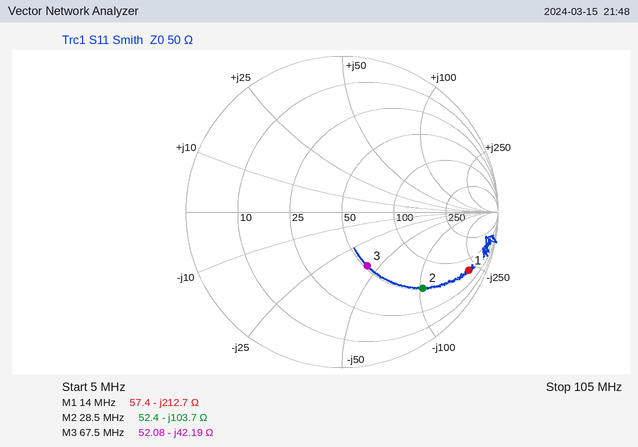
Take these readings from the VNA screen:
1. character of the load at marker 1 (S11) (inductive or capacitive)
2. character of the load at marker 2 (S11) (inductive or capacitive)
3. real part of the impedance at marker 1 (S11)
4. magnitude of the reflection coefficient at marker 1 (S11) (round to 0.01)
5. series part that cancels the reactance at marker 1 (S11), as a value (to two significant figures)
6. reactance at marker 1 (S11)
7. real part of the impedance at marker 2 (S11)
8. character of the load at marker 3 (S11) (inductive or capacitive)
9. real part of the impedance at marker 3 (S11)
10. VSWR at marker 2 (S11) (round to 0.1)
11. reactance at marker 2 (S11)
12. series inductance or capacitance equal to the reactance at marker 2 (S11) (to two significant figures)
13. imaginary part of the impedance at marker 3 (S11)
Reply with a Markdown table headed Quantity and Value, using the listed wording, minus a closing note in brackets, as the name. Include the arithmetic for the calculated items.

| Quantity | Value |
|---|---|
| character of the load at marker 1 (S11) | capacitive |
| character of the load at marker 2 (S11) | capacitive |
| real part of the impedance at marker 1 | 57.4 Ω |
| magnitude of the reflection coefficient at marker 1 (S11) | 0.89 |
| series part that cancels the reactance at marker 1 (S11), as a value | L = 212.7 Ω/(2π × 14 MHz) ≈ 2.4 µH |
| reactance at marker 1 | -212.7 Ω |
| real part of the impedance at marker 2 | 52.4 Ω |
| character of the load at marker 3 (S11) | capacitive |
| real part of the impedance at marker 3 | 52.08 Ω |
| VSWR at marker 2 (S11) | 5.9 |
| reactance at marker 2 | -103.7 Ω |
| series inductance or capacitance equal to the reactance at marker 2 (S11) | C = 1/(2π × 28.5 MHz × 103.7 Ω) ≈ 54 pF |
| imaginary part of the impedance at marker 3 | -42.19 Ω |
